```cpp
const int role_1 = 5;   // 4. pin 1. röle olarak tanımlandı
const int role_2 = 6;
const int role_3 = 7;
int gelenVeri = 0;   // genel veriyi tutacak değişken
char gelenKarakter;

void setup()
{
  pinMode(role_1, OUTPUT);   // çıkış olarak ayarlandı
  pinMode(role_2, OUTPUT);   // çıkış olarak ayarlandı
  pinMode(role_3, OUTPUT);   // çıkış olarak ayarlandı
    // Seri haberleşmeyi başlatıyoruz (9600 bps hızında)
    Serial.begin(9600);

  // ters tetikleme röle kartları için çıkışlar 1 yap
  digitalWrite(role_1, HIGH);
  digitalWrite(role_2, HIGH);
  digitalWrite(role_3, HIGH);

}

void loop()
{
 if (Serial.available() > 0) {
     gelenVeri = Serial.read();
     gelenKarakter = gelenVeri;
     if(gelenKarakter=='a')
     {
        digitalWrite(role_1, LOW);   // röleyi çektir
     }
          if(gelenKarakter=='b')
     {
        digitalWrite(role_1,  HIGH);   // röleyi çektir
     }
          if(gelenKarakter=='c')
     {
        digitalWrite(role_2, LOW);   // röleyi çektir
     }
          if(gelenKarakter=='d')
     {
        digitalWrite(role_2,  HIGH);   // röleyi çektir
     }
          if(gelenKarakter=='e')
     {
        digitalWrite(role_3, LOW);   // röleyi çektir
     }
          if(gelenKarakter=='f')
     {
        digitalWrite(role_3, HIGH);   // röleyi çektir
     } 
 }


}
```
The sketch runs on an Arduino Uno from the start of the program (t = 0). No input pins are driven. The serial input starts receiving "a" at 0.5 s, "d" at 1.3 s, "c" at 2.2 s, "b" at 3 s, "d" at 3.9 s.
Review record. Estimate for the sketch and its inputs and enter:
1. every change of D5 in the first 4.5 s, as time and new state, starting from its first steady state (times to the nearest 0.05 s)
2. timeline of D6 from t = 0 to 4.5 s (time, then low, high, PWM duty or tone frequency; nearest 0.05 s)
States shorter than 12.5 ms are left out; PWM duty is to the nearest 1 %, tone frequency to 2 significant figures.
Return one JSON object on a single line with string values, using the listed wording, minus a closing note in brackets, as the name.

{"every change of D5 in the first 4.5 s, as time and new state, starting from its first steady state": "0 s high; 0.5 s low; 3 s high", "timeline of D6 from t = 0 to 4.5 s": "0 s high; 2.2 s low; 3.9 s high"}
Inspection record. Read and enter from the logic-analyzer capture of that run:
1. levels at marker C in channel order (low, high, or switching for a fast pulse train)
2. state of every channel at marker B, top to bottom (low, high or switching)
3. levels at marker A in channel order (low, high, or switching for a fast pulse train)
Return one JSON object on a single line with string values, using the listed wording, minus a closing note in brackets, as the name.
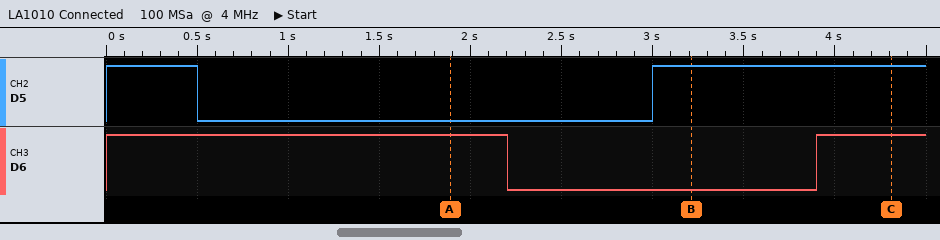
{"levels at marker C in channel order": "D5 high, D6 high", "state of every channel at marker B, top to bottom": "D5 high, D6 low", "levels at marker A in channel order": "D5 low, D6 high"}
